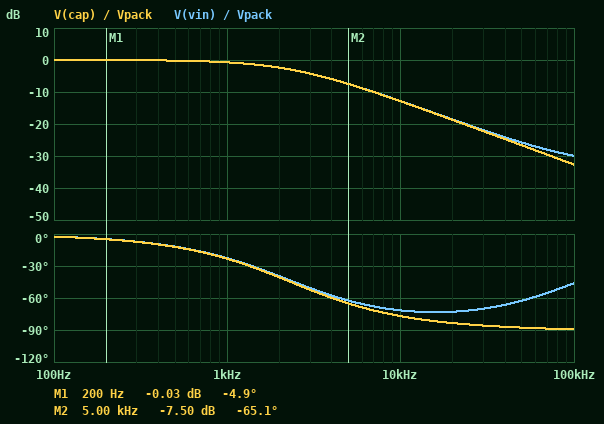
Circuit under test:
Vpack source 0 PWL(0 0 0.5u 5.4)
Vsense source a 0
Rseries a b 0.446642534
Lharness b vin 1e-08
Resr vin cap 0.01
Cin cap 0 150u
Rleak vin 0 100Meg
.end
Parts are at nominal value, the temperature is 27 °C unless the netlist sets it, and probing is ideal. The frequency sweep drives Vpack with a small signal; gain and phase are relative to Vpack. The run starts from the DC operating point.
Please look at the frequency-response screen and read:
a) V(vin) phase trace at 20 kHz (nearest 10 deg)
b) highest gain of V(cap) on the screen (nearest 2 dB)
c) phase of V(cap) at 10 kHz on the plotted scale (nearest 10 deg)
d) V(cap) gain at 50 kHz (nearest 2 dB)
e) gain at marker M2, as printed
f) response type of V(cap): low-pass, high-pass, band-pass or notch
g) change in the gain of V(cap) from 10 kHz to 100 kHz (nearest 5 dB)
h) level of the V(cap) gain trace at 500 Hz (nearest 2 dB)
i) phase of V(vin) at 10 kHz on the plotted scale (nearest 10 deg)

-70 deg
0 dB
-80 deg
-26 dB
-7.50 dB
low-pass
-20 dB
0 dB
-70 deg
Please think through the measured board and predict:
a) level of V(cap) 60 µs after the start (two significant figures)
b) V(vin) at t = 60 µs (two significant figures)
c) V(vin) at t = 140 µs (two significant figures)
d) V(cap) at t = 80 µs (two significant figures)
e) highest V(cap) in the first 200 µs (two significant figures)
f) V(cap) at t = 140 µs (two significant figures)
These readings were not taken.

3.1 V
3.2 V
4.7 V
3.7 V
5.1 V
4.7 V
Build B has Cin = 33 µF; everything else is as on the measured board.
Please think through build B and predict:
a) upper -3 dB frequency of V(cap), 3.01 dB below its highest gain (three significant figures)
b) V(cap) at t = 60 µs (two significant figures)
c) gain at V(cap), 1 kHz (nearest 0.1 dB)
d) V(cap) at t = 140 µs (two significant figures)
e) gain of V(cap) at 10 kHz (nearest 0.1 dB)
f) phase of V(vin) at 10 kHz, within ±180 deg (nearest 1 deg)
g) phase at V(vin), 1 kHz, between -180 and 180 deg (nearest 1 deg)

10.6 kHz
5.3 V
0 dB
5.4 V
-2.8 dB
-42 deg
-5 deg
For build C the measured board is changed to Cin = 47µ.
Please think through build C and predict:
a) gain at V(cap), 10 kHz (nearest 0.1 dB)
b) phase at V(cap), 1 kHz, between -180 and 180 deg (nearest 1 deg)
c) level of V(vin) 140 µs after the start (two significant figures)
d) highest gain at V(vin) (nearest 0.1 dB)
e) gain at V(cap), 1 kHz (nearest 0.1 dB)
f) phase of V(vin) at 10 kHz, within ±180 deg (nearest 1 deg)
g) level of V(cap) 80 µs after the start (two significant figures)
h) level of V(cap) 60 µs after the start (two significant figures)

-4.5 dB
-8 deg
5.4 V
0 dB
-0.1 dB
-52 deg
5.3 V
5.1 V
